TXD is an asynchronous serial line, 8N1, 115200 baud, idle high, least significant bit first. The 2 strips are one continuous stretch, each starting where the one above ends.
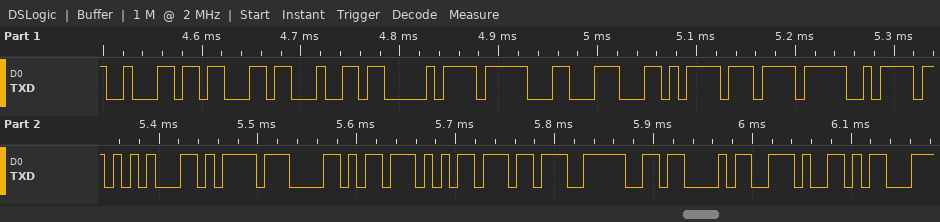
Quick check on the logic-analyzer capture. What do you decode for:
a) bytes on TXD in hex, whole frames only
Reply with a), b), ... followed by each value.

a) 62 63 64 D0 1F 1C BD EF 7A 15 BD 58 57 B7 3E 43 2E 8D
